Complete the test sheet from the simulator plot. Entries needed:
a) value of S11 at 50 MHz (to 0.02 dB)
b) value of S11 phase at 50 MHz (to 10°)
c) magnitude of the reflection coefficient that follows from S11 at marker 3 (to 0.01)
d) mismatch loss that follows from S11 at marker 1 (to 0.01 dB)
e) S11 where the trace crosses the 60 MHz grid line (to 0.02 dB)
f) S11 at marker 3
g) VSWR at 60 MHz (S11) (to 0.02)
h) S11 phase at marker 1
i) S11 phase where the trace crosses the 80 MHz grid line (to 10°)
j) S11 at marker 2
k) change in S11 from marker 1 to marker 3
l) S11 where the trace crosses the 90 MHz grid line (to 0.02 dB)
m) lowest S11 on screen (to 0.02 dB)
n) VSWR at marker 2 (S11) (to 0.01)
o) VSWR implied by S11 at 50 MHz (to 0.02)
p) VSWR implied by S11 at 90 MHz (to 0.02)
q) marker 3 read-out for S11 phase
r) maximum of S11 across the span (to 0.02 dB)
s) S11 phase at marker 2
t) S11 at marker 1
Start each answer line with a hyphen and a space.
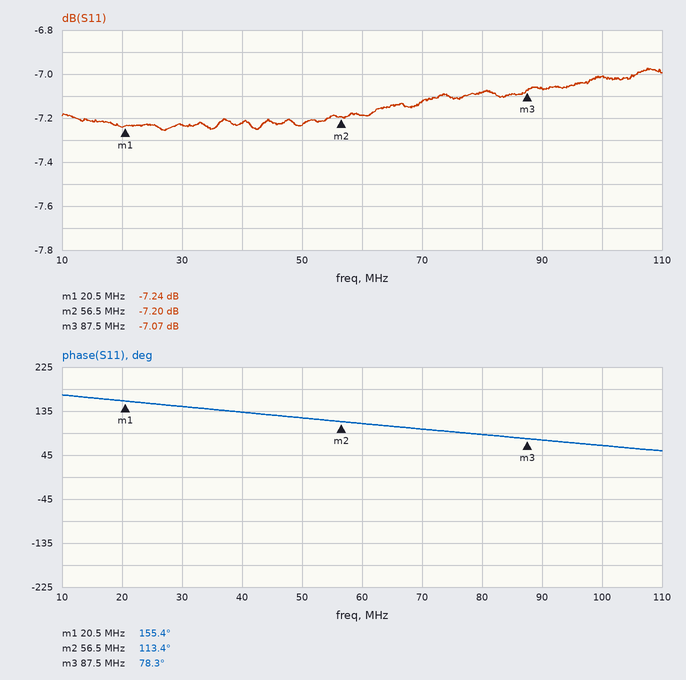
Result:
- -7.24 dB
- 120°
- 0.44
- 0.91 dB
- -7.18 dB
- -7.07 dB
- 2.56
- 155.4°
- 90°
- -7.20 dB
- 0.17 dB
- -7.06 dB
- -7.26 dB
- 2.55
- 2.54
- 2.60
- 78.3°
- -6.98 dB
- 113.4°
- -7.24 dB
